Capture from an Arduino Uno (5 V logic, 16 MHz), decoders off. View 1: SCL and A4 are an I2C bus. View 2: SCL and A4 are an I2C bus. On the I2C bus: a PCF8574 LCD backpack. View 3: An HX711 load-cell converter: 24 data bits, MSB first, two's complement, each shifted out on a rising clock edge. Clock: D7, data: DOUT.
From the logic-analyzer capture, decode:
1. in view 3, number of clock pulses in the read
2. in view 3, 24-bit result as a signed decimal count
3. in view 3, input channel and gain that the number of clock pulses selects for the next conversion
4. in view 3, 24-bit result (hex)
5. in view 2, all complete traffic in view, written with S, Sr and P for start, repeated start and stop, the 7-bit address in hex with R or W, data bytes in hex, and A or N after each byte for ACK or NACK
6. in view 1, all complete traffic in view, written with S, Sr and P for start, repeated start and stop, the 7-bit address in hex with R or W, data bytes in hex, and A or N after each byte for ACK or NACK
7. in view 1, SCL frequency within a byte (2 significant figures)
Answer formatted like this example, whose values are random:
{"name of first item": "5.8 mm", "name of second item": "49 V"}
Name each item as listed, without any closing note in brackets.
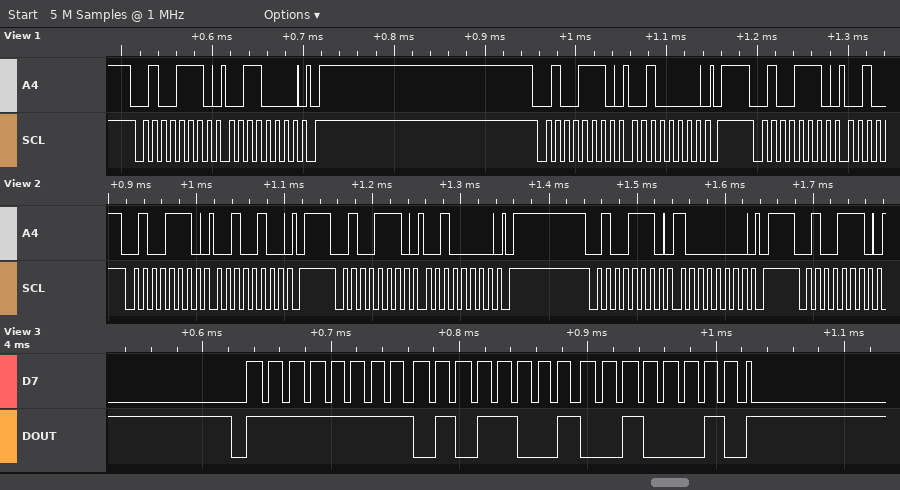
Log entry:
{"in view 3, number of clock pulses in the read": "25", "in view 3, 24-bit result as a signed decimal count": "-42718", "in view 3, input channel and gain that the number of clock pulses selects for the next conversion": "channel A, gain 128", "in view 3, 24-bit result": "0xFF5922", "in view 2, all complete traffic in view, written with S, Sr and P for start, repeated start and stop, the 7-bit address in hex with R or W, data bytes in hex, and A or N after each byte for ACK or NACK": "S 27W A 24 A P S 27W A 20 A P S 27W A 80 A P S 27W A", "in view 1, all complete traffic in view, written with S, Sr and P for start, repeated start and stop, the 7-bit address in hex with R or W, data bytes in hex, and A or N after each byte for ACK or NACK": "S 27W A 30 A P S 27W A 20 A P S 27W A", "in view 1, SCL frequency within a byte": "100 kHz"}
